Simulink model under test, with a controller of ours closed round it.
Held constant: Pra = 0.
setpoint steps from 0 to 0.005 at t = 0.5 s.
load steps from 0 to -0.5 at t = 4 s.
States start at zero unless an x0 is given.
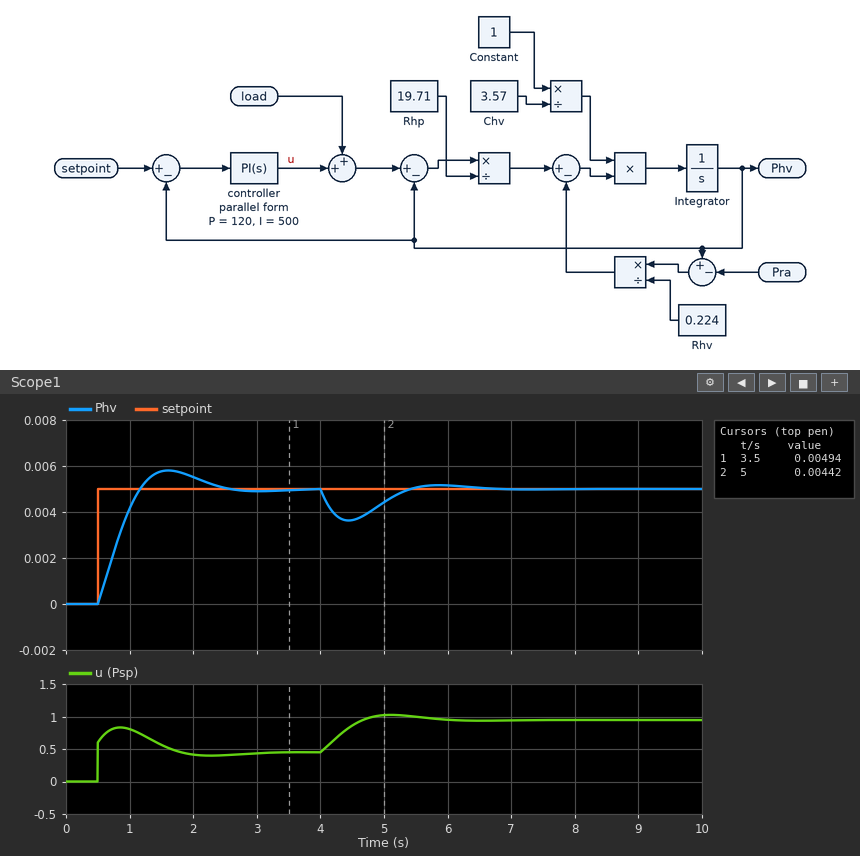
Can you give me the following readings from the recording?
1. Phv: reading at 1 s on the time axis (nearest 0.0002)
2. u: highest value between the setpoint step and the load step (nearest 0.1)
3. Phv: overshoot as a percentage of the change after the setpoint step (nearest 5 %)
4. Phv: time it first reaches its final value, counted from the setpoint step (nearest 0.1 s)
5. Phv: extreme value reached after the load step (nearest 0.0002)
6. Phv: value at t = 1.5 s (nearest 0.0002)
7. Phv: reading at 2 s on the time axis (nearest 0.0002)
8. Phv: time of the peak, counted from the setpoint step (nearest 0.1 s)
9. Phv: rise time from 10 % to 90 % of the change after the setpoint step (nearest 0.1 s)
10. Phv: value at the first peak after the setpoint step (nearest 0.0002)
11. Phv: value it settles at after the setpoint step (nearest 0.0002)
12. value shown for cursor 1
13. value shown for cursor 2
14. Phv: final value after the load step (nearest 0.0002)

0.0042
0.8
15 %
0.7 s
0.0036
0.0058
0.0056
1.1 s
0.5 s
0.0058
0.0050
0.00494
0.00442
0.0050
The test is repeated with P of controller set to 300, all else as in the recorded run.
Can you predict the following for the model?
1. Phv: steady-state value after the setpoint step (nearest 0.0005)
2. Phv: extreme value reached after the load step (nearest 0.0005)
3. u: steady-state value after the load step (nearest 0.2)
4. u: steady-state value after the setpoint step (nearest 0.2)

0.0050
0.0040
1.0
0.4
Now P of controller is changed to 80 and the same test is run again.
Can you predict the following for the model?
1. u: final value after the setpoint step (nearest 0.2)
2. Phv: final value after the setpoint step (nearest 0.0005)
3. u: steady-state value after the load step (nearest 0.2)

0.4
0.0050
1.0
